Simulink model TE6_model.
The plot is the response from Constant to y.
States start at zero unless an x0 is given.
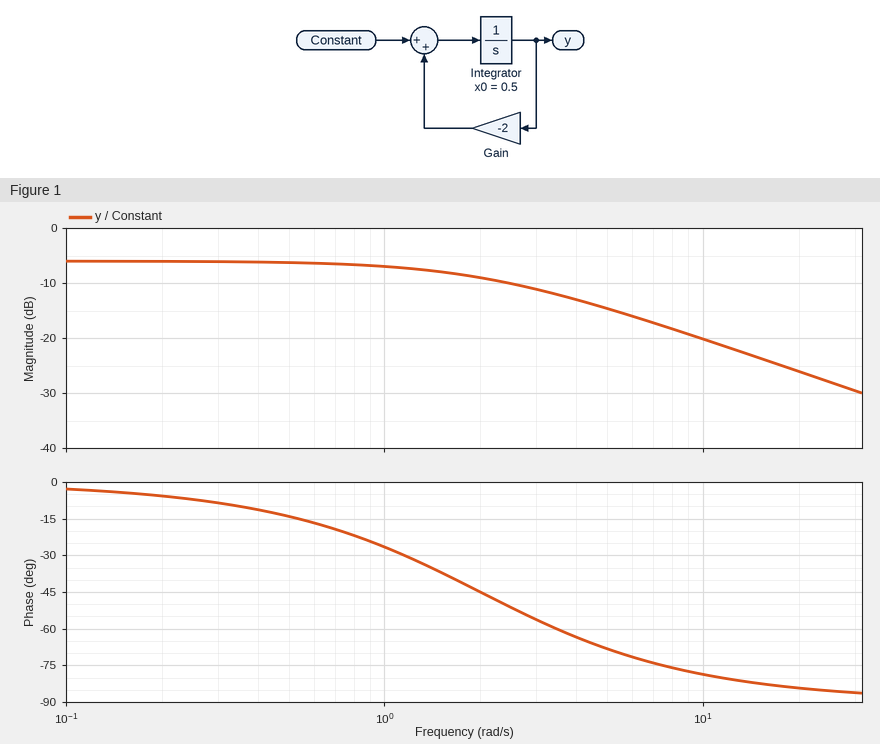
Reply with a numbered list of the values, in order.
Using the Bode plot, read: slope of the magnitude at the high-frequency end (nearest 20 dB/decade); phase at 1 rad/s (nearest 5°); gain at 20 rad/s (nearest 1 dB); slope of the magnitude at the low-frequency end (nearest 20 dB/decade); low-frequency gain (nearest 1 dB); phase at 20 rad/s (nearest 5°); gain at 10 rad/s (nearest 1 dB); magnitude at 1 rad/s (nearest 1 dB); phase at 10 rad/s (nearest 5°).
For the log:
1. -20 dB/decade
2. -25°
3. -26 dB
4. 0 dB/decade
5. -6 dB
6. -85°
7. -20 dB
8. -7 dB
9. -80°
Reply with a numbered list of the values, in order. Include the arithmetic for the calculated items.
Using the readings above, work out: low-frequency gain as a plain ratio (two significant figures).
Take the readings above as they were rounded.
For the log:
1. 10^(-6 / 20) = 0.50
